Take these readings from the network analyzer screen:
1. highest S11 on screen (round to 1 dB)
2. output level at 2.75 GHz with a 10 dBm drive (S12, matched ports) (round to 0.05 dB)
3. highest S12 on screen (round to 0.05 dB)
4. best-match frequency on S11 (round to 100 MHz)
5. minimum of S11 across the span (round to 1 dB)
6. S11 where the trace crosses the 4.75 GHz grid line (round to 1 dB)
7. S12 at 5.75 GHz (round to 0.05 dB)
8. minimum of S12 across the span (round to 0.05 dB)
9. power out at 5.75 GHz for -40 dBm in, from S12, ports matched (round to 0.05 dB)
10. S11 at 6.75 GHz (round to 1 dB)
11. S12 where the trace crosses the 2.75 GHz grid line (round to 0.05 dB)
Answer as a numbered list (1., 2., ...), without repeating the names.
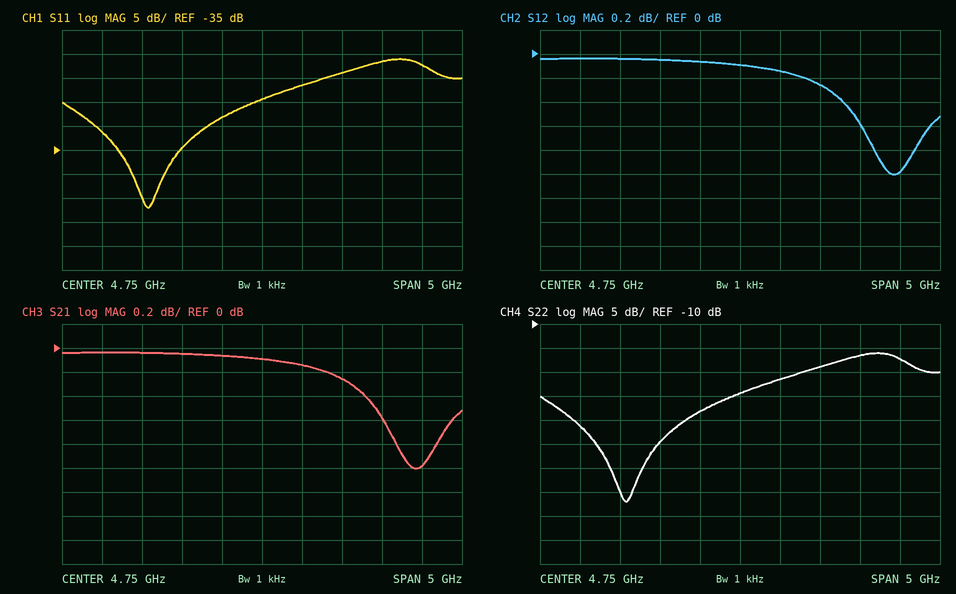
1. -16 dB
2. 9.95 dBm
3. -0.05 dB
4. 3.3 GHz
5. -47 dB
6. -24 dB
7. -0.25 dB
8. -1.00 dB
9. -40.25 dBm
10. -17 dB
11. -0.05 dB
